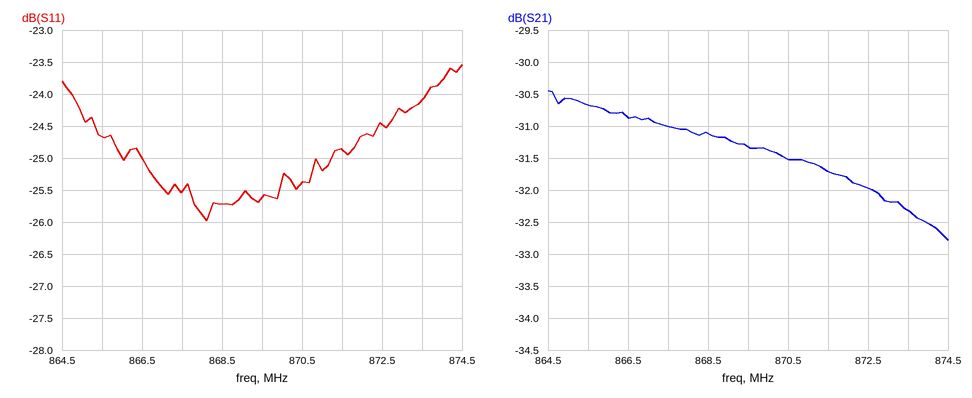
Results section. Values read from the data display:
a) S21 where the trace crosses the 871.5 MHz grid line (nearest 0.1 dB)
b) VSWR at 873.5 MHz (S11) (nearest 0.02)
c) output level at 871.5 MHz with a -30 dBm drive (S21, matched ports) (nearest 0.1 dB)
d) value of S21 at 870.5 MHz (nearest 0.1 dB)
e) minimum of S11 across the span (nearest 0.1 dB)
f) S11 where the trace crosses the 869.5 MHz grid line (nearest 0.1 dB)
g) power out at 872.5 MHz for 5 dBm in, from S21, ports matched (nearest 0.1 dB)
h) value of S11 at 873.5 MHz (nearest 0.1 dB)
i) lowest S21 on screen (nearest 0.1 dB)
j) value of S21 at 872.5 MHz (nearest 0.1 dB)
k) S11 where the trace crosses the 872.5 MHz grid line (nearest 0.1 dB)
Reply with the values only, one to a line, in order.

-31.7 dB
1.14
-61.7 dBm
-31.5 dB
-26.0 dB
-25.6 dB
-27.0 dBm
-24.1 dB
-32.8 dB
-32.0 dB
-24.5 dB
